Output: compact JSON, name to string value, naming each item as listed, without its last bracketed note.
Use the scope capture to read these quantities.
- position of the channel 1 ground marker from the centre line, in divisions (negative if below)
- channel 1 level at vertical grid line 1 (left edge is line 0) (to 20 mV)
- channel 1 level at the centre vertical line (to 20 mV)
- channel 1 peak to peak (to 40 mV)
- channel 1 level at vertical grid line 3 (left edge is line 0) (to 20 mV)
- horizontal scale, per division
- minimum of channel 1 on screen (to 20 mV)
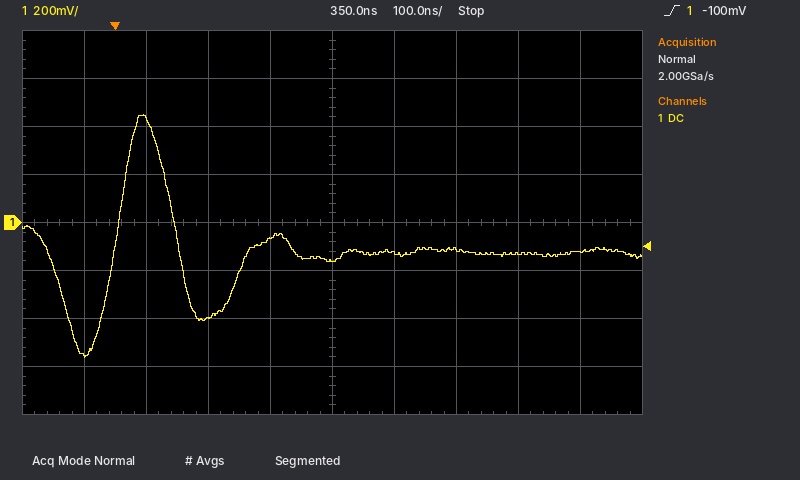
{"position of the channel 1 ground marker from the centre line, in divisions": "0.0 div", "channel 1 level at vertical grid line 1 (left edge is line 0)": "-560 mV", "channel 1 level at the centre vertical line": "-160 mV", "channel 1 peak to peak": "1.00 V", "channel 1 level at vertical grid line 3 (left edge is line 0)": "-400 mV", "horizontal scale, per division": "100 ns", "minimum of channel 1 on screen": "-560 mV"}
